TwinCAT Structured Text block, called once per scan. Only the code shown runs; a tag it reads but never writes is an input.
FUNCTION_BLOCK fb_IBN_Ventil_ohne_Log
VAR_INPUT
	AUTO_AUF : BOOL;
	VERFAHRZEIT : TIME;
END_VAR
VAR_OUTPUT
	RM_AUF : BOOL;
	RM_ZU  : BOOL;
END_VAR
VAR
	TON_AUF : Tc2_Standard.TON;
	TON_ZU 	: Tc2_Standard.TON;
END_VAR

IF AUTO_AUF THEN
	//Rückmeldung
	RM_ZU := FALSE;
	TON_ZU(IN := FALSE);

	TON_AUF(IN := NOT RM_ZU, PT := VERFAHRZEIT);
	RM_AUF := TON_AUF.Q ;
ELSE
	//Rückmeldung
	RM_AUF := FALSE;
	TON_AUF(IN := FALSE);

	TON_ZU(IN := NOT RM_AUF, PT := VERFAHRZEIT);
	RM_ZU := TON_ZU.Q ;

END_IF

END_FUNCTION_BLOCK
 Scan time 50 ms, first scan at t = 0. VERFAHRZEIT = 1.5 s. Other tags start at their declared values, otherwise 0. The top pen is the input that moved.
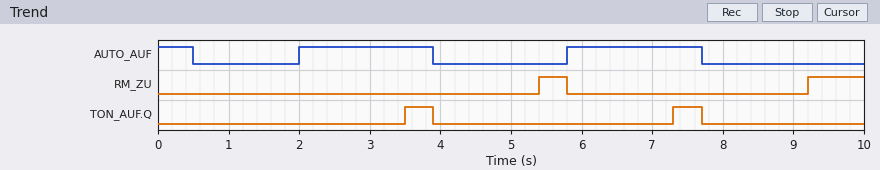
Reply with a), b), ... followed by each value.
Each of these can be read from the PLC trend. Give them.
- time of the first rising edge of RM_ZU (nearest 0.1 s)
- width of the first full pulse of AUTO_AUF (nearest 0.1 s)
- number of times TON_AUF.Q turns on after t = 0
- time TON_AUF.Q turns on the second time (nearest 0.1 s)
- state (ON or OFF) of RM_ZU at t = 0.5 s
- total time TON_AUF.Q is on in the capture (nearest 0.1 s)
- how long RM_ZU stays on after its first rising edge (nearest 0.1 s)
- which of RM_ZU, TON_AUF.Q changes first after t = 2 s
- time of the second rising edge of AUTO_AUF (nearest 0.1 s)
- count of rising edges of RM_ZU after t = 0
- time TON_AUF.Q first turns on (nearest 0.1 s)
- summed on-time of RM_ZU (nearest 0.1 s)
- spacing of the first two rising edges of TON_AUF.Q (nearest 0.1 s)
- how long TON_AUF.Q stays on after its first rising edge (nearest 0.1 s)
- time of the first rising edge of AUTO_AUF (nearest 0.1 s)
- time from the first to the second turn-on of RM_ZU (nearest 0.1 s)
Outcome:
a) 5.4 s
b) 1.9 s
c) 2
d) 7.3 s
e) OFF
f) 0.8 s
g) 0.4 s
h) TON_AUF.Q
i) 5.8 s
j) 2
k) 3.5 s
l) 1.2 s
m) 3.8 s
n) 0.4 s
o) 2.0 s
p) 3.8 s
